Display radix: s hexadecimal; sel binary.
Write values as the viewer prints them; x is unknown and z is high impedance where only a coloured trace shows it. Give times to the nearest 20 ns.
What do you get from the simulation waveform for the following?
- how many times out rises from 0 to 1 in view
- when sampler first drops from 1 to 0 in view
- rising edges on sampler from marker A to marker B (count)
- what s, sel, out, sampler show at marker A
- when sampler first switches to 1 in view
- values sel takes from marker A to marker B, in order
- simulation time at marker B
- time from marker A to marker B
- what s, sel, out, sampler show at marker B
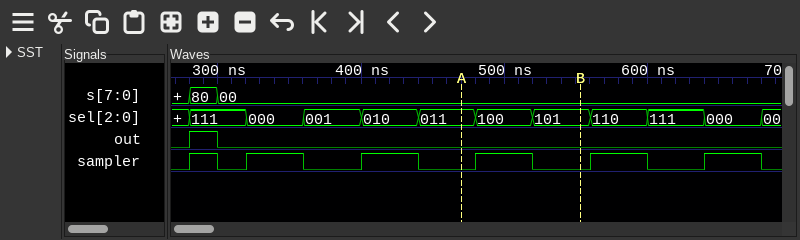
1
300 ns
1
s=00, sel=011, out=0, sampler=0
280 ns
011, 100, 101
560 ns
80 ns
s=00, sel=101, out=0, sampler=0
